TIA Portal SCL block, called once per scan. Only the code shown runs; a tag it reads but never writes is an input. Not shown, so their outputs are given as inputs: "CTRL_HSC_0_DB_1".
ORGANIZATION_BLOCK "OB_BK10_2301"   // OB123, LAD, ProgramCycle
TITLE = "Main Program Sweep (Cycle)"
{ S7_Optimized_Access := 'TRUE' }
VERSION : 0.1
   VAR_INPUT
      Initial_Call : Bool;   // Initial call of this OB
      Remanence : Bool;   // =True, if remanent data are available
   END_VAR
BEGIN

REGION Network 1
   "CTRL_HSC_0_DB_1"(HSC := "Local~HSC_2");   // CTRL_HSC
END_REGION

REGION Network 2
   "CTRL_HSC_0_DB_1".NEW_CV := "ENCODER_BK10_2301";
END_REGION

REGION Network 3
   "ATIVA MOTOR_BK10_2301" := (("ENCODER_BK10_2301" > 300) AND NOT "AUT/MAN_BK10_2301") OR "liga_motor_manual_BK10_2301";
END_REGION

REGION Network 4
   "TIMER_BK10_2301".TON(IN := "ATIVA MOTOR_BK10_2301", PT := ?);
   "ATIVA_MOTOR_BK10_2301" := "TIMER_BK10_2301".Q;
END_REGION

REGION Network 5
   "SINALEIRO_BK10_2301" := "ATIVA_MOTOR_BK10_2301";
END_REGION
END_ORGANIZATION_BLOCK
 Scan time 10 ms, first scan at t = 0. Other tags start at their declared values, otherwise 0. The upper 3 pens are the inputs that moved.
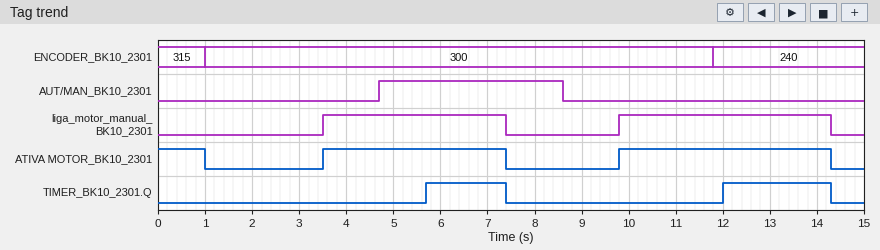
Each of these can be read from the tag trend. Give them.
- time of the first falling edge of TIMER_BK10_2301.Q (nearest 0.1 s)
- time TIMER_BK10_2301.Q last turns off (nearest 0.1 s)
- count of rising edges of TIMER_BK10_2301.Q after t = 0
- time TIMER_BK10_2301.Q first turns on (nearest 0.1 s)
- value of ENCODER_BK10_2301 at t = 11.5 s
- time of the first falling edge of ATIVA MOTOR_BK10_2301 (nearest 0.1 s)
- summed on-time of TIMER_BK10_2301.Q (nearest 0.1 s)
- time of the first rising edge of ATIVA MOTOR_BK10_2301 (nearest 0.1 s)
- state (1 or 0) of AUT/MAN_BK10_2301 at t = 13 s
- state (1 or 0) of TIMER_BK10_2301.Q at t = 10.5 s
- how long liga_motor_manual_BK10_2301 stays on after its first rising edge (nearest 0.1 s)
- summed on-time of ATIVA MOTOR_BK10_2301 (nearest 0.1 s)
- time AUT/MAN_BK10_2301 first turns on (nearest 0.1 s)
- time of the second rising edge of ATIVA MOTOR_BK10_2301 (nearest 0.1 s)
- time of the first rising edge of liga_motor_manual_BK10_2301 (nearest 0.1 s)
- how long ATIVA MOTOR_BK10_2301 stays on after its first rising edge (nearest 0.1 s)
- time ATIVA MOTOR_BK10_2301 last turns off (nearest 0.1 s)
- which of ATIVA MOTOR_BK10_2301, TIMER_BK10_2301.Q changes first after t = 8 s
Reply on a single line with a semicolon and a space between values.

7.4 s; 14.3 s; 2; 5.7 s; 300; 1.0 s; 4.0 s; 3.5 s; 0; 0; 3.9 s; 9.4 s; 4.7 s; 9.8 s; 3.5 s; 3.9 s; 14.3 s; ATIVA MOTOR_BK10_2301
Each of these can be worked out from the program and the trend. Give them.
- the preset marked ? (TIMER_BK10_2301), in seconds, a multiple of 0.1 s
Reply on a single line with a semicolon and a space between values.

2.2 s
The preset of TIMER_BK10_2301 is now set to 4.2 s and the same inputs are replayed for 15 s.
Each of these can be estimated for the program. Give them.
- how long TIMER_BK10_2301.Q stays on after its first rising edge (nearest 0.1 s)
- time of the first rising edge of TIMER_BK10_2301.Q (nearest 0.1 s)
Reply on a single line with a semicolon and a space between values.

0.3 s; 14.0 s
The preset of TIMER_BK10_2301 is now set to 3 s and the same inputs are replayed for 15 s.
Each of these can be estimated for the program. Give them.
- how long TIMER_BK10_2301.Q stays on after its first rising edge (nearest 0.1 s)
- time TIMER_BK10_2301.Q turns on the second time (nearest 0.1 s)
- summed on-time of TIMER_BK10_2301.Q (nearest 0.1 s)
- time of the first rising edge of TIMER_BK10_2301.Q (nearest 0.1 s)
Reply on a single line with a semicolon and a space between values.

0.9 s; 12.8 s; 2.4 s; 6.5 s
